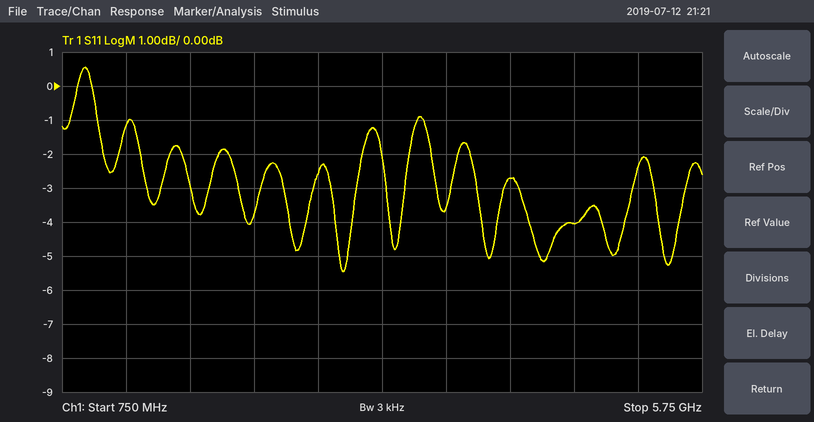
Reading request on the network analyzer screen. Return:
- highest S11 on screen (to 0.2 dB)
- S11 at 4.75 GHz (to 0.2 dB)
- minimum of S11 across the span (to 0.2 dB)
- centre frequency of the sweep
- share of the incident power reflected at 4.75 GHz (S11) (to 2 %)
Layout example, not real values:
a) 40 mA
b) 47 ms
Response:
a) 0.6 dB
b) -4.0 dB
c) -5.4 dB
d) 3.25 GHz
e) 40 %
